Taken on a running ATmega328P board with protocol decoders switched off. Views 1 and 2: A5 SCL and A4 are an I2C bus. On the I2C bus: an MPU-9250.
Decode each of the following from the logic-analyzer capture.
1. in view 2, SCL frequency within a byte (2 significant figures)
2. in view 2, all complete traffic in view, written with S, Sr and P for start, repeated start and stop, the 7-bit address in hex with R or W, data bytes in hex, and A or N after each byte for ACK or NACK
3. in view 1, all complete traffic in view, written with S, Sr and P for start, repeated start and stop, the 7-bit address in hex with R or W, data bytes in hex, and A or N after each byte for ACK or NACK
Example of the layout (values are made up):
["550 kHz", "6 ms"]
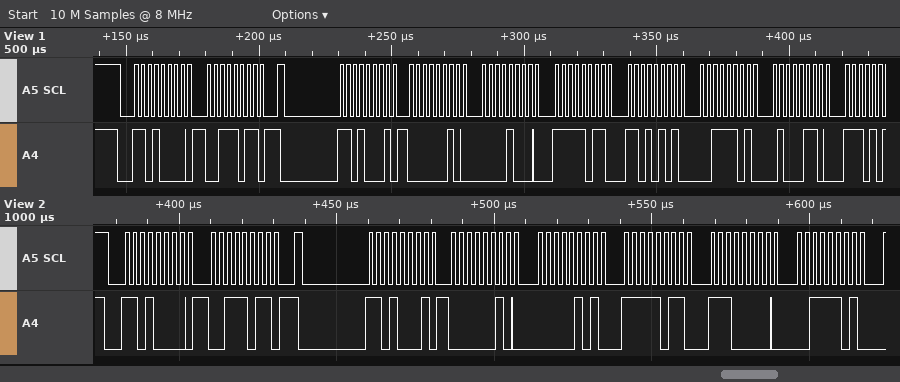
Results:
["400 kHz", "S 68W A 3B A Sr 68R A 02 A 05 A FB A E0 A 3D A", "S 68W A 3B A Sr 68R A 02 A 08 A FB A D5 A 3D A 46 A"]
